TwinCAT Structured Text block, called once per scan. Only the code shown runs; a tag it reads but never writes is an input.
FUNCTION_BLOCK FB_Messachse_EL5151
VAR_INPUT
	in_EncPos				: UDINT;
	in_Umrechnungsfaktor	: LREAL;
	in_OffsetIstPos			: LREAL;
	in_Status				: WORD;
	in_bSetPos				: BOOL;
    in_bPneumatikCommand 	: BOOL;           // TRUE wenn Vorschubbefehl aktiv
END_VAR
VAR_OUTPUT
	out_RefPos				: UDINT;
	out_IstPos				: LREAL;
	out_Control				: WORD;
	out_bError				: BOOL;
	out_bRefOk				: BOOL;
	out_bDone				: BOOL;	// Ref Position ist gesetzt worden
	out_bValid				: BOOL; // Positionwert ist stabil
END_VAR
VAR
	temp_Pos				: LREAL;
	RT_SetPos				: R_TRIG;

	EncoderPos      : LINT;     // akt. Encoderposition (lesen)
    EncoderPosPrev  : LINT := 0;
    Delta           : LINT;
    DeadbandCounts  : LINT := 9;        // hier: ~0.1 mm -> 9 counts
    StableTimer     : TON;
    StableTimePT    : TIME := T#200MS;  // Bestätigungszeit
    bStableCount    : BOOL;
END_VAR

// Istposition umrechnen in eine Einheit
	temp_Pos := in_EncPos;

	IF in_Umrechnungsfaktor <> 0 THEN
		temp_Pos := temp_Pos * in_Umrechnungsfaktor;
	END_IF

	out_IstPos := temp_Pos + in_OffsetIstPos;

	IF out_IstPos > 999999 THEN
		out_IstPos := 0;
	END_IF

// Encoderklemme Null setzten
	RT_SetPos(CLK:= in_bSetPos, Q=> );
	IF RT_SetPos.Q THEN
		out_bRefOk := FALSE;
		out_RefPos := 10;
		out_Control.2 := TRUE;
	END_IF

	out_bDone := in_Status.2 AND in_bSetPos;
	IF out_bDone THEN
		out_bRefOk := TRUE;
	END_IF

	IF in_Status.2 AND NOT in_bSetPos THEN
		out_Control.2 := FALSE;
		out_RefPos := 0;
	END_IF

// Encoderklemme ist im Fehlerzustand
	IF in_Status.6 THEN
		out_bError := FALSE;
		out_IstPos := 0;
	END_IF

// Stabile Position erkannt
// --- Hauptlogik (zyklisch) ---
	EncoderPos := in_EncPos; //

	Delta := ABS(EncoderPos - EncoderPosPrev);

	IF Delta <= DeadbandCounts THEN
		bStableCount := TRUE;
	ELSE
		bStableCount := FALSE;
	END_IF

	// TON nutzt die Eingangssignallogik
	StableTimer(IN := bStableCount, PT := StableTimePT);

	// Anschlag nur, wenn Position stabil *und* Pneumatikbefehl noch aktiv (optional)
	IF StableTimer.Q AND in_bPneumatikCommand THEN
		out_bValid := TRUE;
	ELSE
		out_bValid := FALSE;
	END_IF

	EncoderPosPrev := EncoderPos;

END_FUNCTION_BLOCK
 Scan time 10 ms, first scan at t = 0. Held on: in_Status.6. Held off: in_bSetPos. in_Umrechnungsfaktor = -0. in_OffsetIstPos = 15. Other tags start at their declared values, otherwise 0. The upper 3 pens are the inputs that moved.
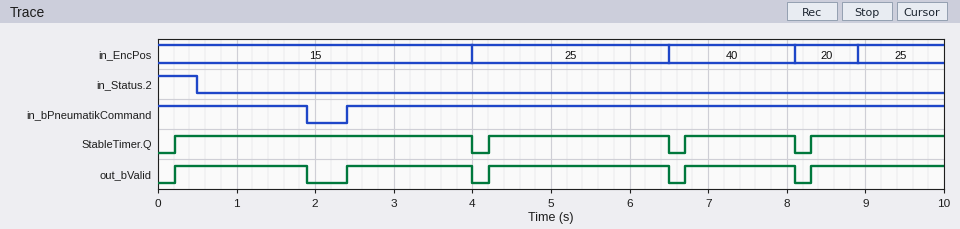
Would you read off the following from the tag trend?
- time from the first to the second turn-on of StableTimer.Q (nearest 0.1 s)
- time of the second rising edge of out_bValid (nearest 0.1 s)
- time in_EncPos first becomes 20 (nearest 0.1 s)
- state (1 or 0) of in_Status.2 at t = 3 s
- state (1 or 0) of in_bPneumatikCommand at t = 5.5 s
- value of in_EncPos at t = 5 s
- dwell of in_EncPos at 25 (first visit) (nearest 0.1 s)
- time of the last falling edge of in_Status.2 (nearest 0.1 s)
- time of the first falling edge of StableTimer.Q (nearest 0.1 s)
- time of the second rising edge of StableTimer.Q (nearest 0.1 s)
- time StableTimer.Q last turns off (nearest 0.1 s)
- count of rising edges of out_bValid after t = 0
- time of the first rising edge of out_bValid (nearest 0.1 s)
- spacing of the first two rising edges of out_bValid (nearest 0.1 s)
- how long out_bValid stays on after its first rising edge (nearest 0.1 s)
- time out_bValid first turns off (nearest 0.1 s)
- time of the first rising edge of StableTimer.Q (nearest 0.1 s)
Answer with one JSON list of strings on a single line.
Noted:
["4.0 s", "2.4 s", "8.1 s", "0", "1", "25", "2.5 s", "0.5 s", "4.0 s", "4.2 s", "8.1 s", "5", "0.2 s", "2.2 s", "1.7 s", "1.9 s", "0.2 s"]
